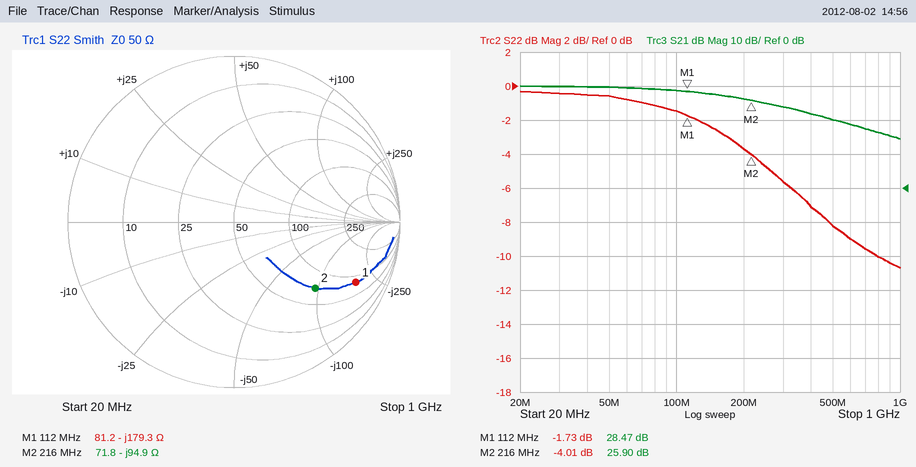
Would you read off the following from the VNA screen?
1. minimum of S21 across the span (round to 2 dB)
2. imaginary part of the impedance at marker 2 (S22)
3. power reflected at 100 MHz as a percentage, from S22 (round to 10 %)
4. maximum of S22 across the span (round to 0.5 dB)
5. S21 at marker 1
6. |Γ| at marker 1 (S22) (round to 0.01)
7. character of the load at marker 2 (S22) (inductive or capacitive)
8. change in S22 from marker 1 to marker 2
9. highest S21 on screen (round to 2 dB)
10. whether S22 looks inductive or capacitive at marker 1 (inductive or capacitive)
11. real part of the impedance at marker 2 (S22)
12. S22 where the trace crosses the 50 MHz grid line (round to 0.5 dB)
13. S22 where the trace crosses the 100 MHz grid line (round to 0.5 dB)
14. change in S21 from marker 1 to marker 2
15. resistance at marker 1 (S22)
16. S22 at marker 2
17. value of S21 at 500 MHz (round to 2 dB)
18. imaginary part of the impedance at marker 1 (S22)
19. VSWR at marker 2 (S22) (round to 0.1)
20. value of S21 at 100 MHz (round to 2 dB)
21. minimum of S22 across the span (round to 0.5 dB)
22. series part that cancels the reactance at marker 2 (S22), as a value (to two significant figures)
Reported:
14 dB
-94.9 Ω
70 %
-0.5 dB
28.47 dB
0.82
capacitive
-2.28 dB
30 dB
capacitive
71.8 Ω
-0.5 dB
-1.5 dB
-2.57 dB
81.2 Ω
-4.01 dB
20 dB
-179.3 Ω
4.4
28 dB
-10.5 dB
70 nH
